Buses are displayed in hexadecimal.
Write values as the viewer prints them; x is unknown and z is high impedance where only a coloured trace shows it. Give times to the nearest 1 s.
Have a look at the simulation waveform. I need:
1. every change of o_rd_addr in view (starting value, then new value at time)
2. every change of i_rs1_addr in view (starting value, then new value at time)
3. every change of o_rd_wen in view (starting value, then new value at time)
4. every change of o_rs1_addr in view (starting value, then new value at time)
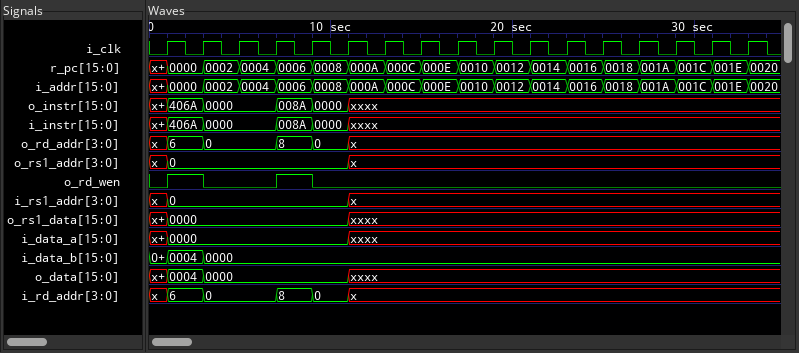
x, 6 at 1 s, 0 at 3 s, 8 at 7 s, 0 at 9 s, x at 11 s
x, 0 at 1 s, x at 11 s
0, 1 at 1 s, 0 at 3 s, 1 at 7 s, 0 at 9 s
x, 0 at 1 s, x at 11 s
